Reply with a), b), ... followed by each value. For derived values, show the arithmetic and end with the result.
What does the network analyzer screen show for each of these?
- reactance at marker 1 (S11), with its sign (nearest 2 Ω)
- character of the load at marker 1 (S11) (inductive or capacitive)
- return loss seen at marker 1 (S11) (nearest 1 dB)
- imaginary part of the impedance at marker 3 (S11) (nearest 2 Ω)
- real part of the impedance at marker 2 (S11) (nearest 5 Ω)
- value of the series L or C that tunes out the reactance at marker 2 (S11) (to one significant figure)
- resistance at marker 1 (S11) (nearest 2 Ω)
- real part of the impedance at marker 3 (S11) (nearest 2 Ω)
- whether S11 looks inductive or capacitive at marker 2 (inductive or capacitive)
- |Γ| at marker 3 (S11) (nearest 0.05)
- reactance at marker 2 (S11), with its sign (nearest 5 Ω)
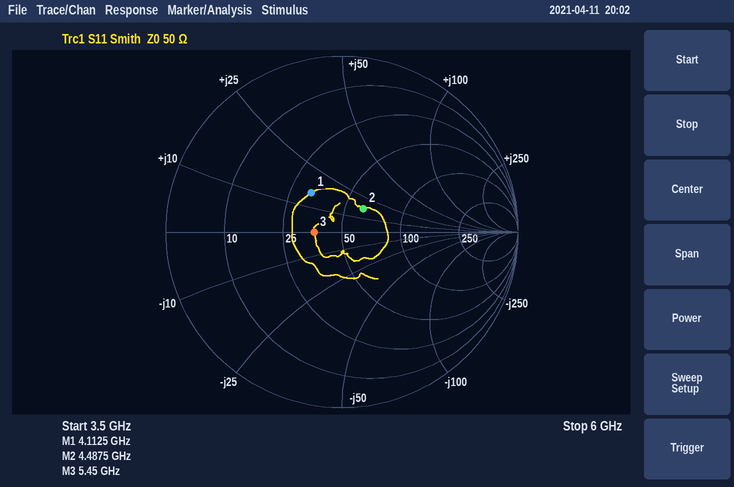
a) +16 Ω
b) inductive
c) 11 dB
d) 0 Ω
e) 60 Ω
f) C = 1/(2π × 4.4875 GHz × 15 Ω) ≈ 2 pF
g) 32 Ω
h) 36 Ω
i) inductive
j) 0.15
k) +15 Ω
